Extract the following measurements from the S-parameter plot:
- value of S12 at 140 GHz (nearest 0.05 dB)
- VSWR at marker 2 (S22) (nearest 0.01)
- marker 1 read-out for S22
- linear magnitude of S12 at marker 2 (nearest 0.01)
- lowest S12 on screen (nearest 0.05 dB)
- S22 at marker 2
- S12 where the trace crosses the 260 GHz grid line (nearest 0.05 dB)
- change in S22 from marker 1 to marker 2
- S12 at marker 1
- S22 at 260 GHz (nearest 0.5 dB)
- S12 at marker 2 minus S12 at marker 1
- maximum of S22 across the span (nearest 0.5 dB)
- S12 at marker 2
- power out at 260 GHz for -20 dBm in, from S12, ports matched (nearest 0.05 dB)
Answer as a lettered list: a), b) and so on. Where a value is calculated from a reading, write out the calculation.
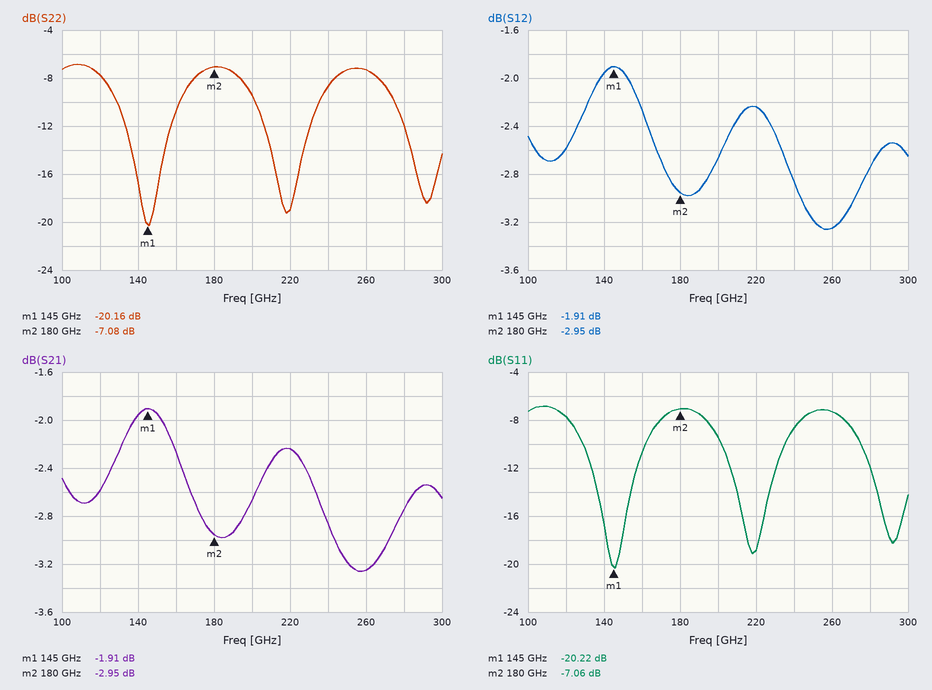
a) -1.95 dB
b) (1 + 0.4426)/(1 − 0.4426) ≈ 2.59
c) -20.16 dB
d) 10^(-2.95/20) ≈ 0.71
e) -3.25 dB
f) -7.08 dB
g) -3.25 dB
h) -7.08 − (-20.16) = 13.08 dB
i) -1.91 dB
j) -7.5 dB
k) -2.95 − (-1.91) = -1.04 dB
l) -7.0 dB
m) -2.95 dB
n) -20 dBm + (-3.25 dB) = -23.25 dBm
